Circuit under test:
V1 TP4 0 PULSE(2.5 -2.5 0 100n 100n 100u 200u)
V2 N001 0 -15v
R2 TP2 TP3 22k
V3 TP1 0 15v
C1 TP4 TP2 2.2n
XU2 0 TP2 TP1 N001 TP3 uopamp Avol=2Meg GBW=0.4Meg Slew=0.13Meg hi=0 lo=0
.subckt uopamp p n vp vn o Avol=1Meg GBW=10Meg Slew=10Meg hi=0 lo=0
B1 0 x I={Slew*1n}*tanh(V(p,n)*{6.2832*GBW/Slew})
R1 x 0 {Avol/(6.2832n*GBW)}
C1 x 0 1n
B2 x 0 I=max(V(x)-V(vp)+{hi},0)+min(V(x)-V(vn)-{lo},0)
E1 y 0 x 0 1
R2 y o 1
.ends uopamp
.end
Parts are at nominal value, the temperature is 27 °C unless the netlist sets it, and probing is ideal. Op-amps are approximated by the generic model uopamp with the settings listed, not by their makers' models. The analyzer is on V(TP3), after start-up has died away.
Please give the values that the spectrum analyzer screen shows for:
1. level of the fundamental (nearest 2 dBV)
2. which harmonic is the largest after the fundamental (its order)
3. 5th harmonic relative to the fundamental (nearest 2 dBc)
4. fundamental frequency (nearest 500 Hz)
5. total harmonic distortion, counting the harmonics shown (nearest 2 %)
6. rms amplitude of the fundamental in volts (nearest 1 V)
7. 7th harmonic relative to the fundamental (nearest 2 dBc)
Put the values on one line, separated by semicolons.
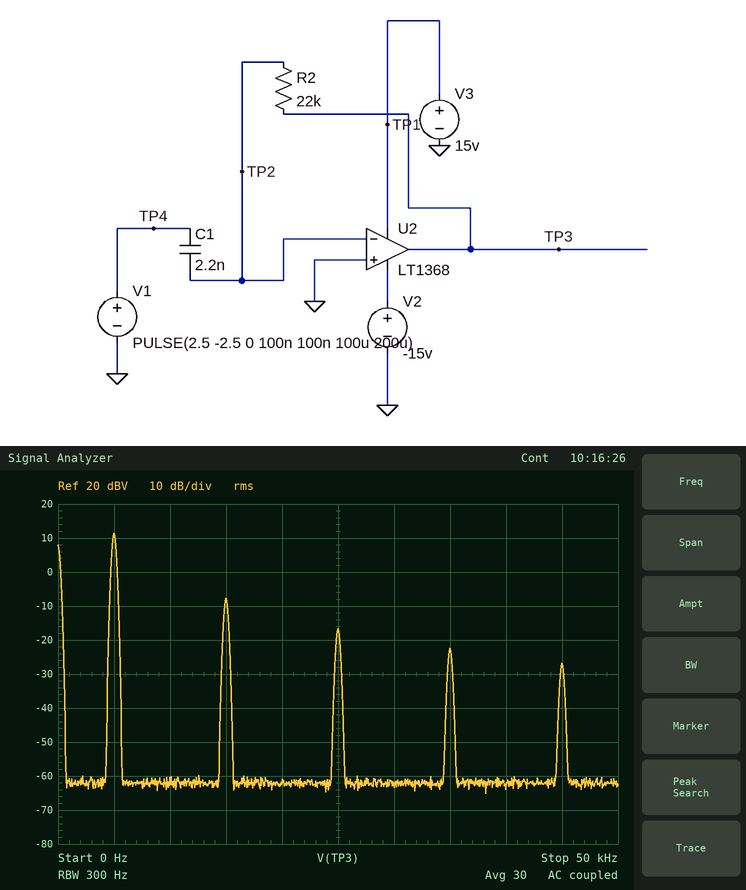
12 dBV; 3; -28 dBc; 5.0 kHz; 12 %; 4 V; -34 dBc
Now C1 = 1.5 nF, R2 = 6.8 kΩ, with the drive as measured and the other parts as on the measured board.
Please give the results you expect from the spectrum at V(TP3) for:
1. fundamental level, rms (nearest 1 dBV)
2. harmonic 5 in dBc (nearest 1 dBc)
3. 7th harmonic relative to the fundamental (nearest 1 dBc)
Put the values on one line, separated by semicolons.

-8 dBV; -1 dBc; -8 dBc
